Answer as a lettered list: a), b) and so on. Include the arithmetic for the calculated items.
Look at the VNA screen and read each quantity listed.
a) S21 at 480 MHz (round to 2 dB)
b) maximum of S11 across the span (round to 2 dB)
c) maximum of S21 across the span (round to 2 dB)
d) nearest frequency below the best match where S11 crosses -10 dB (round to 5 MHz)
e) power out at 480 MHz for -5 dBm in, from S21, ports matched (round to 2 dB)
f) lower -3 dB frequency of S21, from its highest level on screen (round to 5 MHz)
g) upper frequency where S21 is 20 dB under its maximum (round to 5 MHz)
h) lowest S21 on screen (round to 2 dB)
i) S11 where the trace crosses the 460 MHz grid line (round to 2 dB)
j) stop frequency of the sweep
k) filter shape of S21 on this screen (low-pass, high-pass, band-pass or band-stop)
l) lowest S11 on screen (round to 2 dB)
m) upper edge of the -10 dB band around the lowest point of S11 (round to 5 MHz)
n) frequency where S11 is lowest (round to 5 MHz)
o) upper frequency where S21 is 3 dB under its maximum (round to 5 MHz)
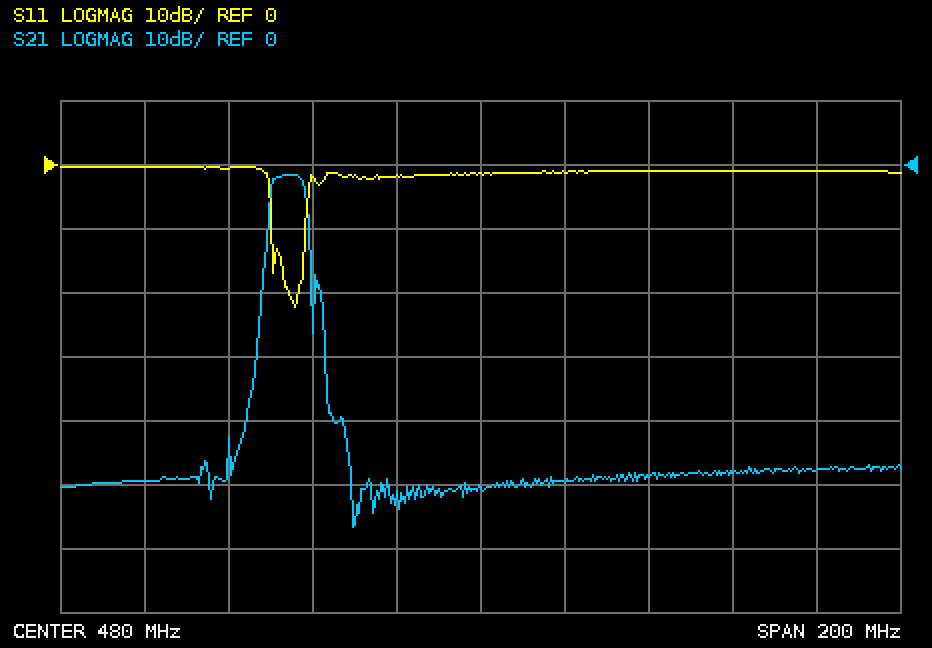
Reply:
a) -50 dB
b) 0 dB
c) -2 dB
d) 430 MHz
e) -5 dBm + (-50 dB) = -56 dBm
f) 430 MHz
g) 440 MHz
h) -56 dB
i) -2 dB
j) 580 MHz
k) band-pass
l) -22 dB
m) 440 MHz
n) 435 MHz
o) 440 MHz
